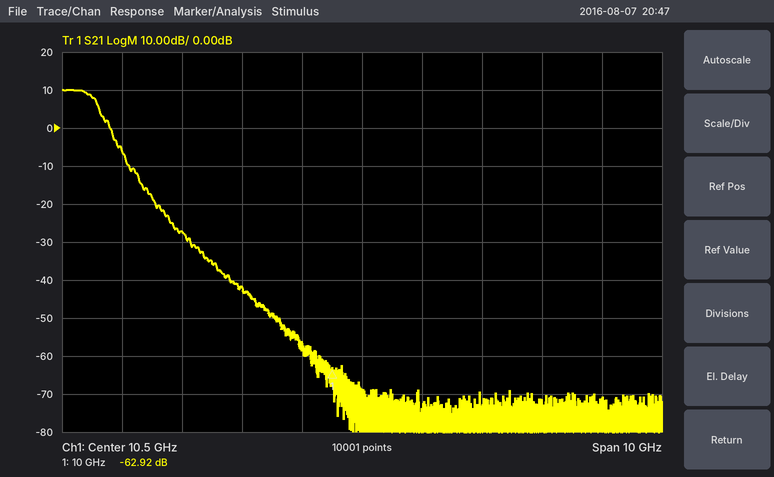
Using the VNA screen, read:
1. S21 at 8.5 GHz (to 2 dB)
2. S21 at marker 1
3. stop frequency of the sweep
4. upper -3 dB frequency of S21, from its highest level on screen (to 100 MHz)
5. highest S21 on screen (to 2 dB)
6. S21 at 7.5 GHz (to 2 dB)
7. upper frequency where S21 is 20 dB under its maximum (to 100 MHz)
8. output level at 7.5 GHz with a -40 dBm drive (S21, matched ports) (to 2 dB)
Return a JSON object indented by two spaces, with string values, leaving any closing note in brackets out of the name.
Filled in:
{
  "S21 at 8.5 GHz": "-42 dB",
  "S21 at marker 1": "-62.92 dB",
  "stop frequency of the sweep": "15.5 GHz",
  "upper -3 dB frequency of S21, from its highest level on screen": "6.1 GHz",
  "highest S21 on screen": "10 dB",
  "S21 at 7.5 GHz": "-28 dB",
  "upper frequency where S21 is 20 dB under its maximum": "6.6 GHz",
  "output level at 7.5 GHz with a -40 dBm drive (S21, matched ports)": "-68 dBm"
}
